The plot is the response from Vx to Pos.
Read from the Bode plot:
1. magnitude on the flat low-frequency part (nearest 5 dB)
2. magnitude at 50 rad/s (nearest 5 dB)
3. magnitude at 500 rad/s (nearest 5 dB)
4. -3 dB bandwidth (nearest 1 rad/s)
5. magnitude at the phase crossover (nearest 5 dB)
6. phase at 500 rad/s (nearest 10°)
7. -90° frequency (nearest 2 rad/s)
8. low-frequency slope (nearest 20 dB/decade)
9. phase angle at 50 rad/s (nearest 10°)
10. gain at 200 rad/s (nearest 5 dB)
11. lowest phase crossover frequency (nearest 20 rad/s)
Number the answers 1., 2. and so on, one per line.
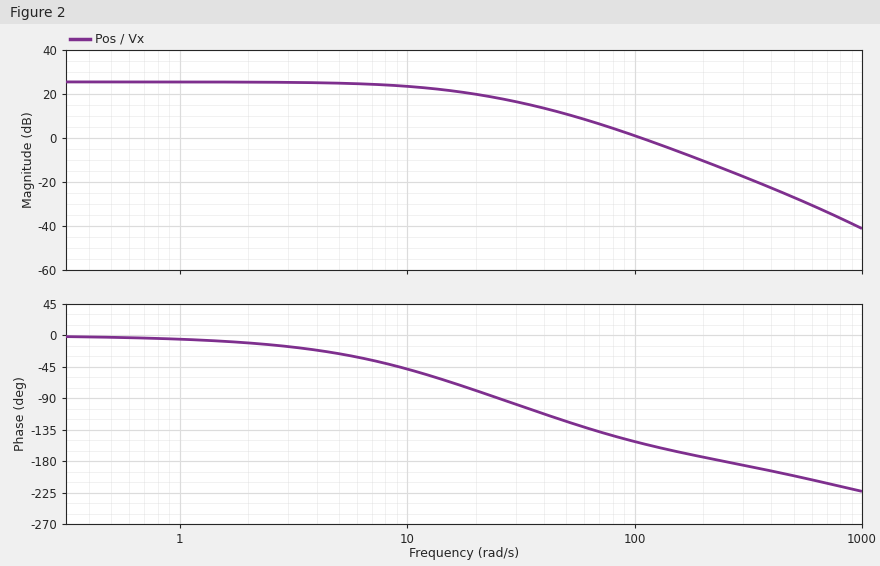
1. 25 dB
2. 10 dB
3. -25 dB
4. 13 rad/s
5. -15 dB
6. -200°
7. 26 rad/s
8. 0 dB/decade
9. -120°
10. -10 dB
11. 240 rad/s
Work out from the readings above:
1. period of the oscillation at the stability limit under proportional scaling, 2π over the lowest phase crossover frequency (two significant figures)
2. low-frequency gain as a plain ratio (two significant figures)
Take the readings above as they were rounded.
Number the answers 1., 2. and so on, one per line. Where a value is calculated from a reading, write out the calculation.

1. 2π / 240 = 0.026 s
2. 10^(25 / 20) = 18
